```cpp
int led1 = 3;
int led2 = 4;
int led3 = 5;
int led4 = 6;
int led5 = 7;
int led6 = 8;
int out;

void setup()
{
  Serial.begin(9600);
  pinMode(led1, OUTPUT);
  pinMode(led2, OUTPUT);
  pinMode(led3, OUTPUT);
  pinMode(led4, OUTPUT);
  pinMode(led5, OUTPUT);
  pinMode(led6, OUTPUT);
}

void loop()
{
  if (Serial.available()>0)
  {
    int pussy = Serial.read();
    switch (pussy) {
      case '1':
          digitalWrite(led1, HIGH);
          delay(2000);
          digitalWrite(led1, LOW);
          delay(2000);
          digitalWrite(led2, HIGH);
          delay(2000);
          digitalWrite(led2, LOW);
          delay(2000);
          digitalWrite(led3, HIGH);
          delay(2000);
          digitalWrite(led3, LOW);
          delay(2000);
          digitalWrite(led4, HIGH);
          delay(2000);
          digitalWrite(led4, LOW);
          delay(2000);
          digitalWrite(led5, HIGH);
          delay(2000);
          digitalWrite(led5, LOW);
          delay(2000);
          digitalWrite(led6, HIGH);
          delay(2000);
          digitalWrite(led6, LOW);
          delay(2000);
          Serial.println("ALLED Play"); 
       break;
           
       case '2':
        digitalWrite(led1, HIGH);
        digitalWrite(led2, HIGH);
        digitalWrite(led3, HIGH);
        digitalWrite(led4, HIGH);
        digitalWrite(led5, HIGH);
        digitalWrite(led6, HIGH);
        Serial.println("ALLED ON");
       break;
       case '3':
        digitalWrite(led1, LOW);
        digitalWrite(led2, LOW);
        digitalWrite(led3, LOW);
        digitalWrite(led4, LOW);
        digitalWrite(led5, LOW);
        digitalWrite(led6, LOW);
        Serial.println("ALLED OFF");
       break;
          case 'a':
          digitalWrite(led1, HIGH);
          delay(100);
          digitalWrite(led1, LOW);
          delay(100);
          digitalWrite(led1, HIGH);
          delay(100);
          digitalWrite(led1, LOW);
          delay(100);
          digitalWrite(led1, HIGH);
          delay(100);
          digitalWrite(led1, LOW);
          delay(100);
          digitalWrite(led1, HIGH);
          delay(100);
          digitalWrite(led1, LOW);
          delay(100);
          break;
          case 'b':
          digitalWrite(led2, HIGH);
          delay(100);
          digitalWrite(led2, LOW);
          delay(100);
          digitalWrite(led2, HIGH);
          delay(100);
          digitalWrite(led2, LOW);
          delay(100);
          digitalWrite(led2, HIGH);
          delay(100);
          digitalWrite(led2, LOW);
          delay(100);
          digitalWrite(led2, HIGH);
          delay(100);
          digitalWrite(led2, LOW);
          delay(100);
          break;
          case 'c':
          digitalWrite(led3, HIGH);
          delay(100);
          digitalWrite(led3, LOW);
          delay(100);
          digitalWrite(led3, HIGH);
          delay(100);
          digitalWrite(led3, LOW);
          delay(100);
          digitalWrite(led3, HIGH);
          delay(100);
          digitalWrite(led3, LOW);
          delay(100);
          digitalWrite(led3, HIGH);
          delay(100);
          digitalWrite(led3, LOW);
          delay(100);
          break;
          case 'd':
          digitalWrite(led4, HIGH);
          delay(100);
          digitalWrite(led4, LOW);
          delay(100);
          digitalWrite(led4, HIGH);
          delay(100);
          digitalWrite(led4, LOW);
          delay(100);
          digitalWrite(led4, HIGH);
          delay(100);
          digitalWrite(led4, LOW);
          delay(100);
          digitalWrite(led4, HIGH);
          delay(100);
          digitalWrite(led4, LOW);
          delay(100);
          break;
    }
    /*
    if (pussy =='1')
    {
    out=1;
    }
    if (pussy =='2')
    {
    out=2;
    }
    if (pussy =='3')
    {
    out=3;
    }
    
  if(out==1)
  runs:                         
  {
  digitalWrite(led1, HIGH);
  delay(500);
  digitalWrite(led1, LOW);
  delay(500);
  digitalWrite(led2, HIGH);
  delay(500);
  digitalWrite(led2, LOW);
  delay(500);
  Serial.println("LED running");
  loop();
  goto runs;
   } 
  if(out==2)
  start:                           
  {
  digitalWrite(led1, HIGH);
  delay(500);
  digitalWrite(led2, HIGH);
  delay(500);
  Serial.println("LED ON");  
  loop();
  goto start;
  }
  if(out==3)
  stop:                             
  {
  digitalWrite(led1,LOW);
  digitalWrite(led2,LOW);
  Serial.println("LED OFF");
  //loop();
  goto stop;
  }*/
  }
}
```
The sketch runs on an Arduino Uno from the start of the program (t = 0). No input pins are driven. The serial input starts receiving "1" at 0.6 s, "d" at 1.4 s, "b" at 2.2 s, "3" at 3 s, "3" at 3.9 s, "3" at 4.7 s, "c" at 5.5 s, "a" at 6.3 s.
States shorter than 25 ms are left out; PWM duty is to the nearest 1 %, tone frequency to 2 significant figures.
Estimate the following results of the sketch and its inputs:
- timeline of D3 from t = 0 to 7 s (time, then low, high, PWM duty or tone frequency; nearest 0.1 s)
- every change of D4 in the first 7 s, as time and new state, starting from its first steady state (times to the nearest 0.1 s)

0 s low; 0.6 s high; 2.6 s low
0 s low; 4.6 s high; 6.6 s low
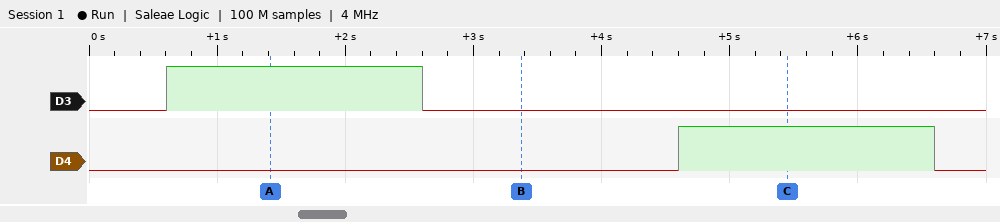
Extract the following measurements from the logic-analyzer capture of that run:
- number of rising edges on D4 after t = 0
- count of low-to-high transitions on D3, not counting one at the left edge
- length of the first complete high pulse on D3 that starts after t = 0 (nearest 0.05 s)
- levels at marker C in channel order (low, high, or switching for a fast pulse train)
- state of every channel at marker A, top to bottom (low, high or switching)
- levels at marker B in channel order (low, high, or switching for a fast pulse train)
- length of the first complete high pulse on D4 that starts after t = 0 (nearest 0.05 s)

1
1
2.00 s
D3 low, D4 high
D3 high, D4 low
D3 low, D4 low
2.00 s
